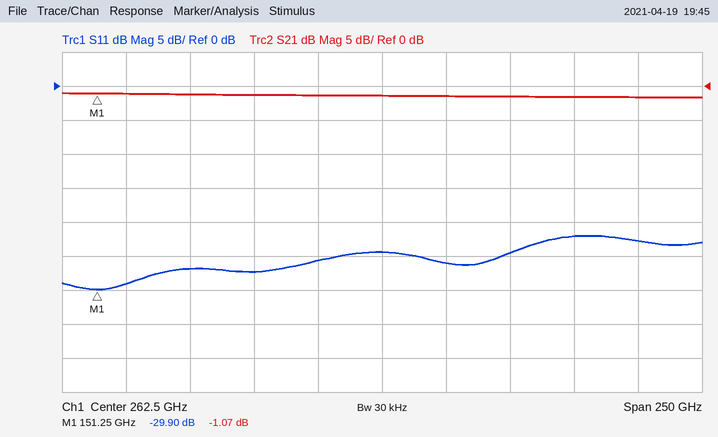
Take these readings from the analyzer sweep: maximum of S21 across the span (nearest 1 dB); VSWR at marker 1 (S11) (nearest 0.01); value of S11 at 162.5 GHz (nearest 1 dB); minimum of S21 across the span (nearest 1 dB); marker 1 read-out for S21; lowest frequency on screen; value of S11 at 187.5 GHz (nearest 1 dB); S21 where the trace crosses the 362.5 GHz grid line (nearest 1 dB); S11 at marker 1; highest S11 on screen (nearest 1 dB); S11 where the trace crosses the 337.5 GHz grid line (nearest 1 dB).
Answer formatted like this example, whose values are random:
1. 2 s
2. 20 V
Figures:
1. -1 dB
2. 1.07
3. -29 dB
4. -2 dB
5. -1.07 dB
6. 137.5 GHz
7. -27 dB
8. -2 dB
9. -29.90 dB
10. -22 dB
11. -22 dB
